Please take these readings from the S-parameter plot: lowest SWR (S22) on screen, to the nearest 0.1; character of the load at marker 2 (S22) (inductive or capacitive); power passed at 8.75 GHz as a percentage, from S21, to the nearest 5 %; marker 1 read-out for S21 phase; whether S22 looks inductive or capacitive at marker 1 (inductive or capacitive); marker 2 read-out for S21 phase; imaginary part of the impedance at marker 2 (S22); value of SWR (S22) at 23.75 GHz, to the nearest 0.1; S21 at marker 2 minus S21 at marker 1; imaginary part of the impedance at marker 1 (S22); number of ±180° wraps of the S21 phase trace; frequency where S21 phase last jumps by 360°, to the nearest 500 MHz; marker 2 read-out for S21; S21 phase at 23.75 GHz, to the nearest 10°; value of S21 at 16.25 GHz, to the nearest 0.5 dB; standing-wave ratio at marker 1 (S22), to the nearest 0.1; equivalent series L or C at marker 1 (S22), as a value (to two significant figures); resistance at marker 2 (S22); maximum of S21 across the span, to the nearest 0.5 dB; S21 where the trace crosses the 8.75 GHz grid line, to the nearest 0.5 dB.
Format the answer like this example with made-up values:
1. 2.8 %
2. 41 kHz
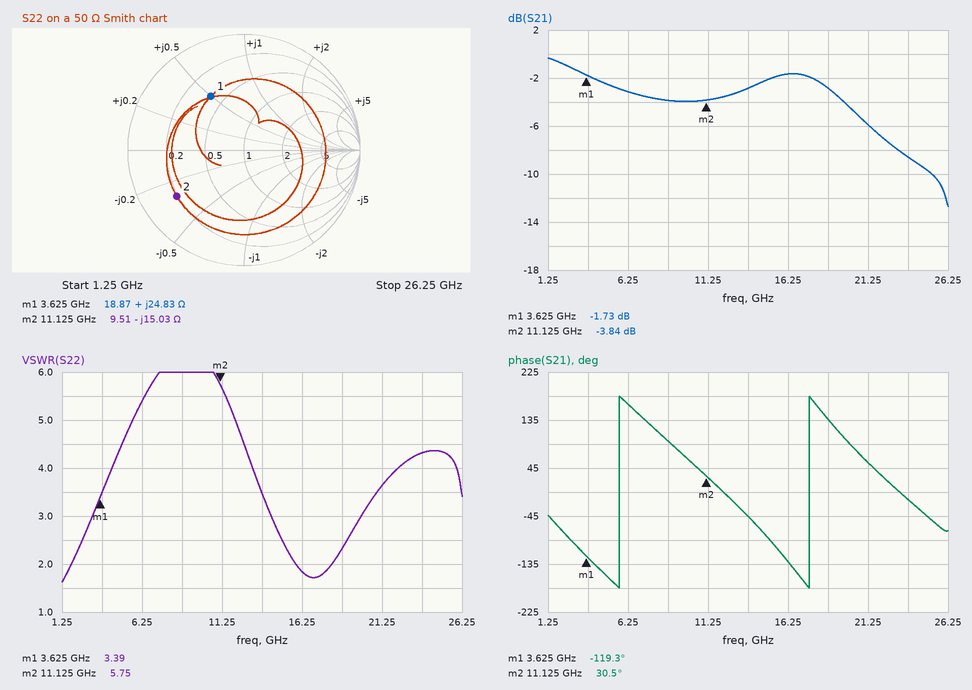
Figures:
1. 1.6
2. capacitive
3. 40 %
4. -119.3°
5. inductive
6. 30.5°
7. -15.03 Ω
8. 4.3
9. -2.11 dB
10. +24.83 Ω
11. 2
12. 17.5 GHz
13. -3.84 dB
14. -10°
15. -1.5 dB
16. 3.4
17. 1.1 nH
18. 9.51 Ω
19. -0.5 dB
20. -4.0 dB
